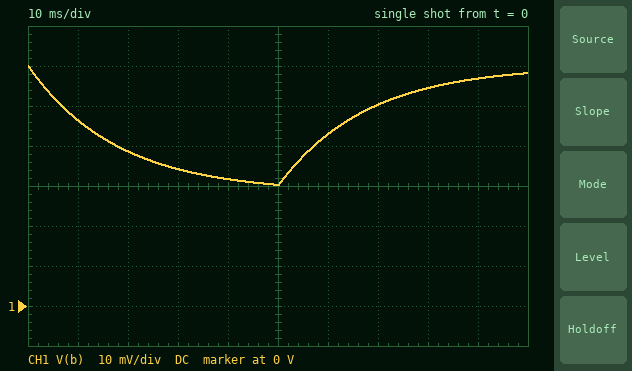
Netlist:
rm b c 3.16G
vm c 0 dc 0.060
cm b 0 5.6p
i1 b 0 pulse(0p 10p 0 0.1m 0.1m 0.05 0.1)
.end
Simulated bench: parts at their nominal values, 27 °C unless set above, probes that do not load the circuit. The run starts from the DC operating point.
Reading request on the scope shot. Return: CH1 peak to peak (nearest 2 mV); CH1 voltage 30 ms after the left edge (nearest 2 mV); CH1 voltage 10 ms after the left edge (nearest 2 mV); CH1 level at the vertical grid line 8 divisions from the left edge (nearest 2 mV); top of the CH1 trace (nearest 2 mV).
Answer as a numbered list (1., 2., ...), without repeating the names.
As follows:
1. 30 mV
2. 34 mV
3. 46 mV
4. 54 mV
5. 60 mV
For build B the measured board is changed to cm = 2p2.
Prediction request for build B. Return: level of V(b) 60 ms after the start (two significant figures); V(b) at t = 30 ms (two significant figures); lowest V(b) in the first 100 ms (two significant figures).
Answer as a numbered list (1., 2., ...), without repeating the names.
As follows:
1. 52 mV
2. 29 mV
3. 28 mV
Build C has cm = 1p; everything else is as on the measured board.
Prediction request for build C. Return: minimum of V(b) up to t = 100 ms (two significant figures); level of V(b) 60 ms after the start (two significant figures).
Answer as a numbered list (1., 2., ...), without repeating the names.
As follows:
1. 28 mV
2. 59 mV
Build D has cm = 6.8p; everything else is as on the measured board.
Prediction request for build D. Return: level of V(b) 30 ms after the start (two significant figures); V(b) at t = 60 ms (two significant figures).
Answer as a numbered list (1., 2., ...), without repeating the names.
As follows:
1. 36 mV
2. 42 mV
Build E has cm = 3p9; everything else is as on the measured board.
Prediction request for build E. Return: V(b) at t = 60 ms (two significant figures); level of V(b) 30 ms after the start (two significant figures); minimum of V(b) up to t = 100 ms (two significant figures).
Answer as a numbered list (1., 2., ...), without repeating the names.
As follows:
1. 46 mV
2. 31 mV
3. 29 mV
